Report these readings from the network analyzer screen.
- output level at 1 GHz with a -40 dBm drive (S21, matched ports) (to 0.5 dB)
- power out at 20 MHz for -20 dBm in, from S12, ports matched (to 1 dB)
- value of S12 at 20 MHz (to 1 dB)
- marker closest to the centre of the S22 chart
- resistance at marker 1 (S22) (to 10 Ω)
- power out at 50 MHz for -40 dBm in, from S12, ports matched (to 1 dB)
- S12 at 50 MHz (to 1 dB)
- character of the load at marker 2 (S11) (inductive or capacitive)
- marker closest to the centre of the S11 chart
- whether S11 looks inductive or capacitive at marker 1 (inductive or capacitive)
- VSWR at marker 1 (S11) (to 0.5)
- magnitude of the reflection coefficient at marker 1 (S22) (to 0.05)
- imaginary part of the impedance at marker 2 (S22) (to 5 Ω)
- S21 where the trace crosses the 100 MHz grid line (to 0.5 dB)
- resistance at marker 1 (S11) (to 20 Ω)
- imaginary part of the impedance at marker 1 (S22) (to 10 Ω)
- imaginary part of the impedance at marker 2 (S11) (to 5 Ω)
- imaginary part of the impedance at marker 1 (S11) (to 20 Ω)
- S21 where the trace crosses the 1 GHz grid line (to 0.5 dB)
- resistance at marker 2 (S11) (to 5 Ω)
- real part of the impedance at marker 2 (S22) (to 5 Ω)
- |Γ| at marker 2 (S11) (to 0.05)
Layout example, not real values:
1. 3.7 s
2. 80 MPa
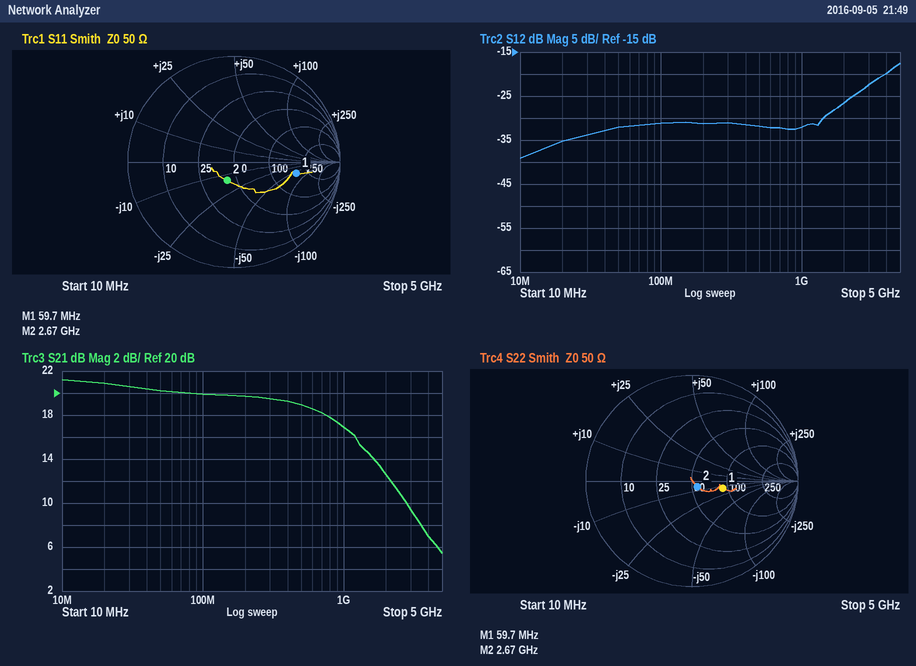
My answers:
1. -23.0 dBm
2. -55 dBm
3. -35 dB
4. marker 2
5. 90 Ω
6. -72 dBm
7. -32 dB
8. capacitive
9. marker 2
10. capacitive
11. 4.0
12. 0.30
13. -5 Ω
14. 20.0 dB
15. 180 Ω
16. -10 Ω
17. -15 Ω
18. -60 Ω
19. 17.0 dB
20. 40 Ω
21. 55 Ω
22. 0.20
